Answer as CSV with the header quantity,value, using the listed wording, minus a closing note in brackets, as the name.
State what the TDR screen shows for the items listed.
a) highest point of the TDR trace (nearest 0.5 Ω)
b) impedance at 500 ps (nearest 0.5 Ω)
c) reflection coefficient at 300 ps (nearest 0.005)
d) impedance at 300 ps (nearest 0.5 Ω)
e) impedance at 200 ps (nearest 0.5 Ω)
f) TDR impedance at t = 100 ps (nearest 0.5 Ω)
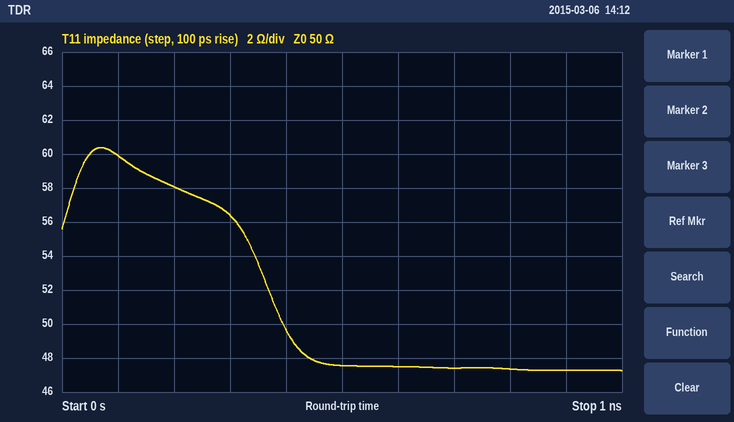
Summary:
quantity,value
highest point of the TDR trace,60.5 Ω
impedance at 500 ps,47.5 Ω
reflection coefficient at 300 ps,+0.060
impedance at 300 ps,56.5 Ω
impedance at 200 ps,58.0 Ω
TDR impedance at t = 100 ps,60.0 Ω
